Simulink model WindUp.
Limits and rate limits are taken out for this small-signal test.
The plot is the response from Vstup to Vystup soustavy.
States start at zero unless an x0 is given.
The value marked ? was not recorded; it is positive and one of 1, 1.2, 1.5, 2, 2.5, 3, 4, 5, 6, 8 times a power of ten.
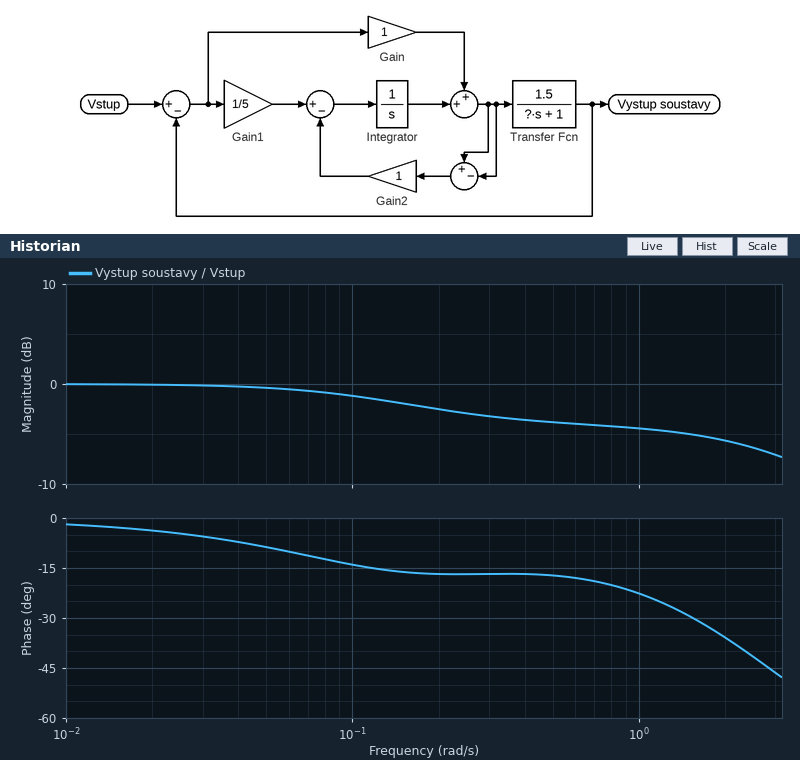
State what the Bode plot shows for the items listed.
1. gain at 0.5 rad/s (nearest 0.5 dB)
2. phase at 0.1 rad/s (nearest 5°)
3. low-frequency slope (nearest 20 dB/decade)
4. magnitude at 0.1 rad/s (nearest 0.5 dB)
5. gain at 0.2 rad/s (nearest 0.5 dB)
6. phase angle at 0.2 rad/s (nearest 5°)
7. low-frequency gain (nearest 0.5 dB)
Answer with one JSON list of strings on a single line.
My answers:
["-4.0 dB", "-15°", "0 dB/decade", "-1.0 dB", "-2.5 dB", "-15°", "0.0 dB"]
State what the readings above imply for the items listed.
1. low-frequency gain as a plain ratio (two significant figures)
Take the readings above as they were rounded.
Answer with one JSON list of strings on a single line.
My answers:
["1.0"]
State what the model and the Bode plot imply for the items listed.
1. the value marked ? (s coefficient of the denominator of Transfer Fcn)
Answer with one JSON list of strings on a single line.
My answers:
["0.8"]
